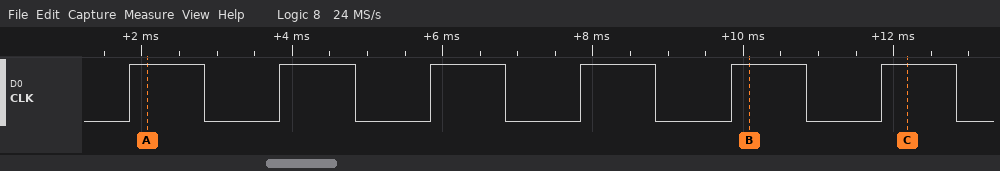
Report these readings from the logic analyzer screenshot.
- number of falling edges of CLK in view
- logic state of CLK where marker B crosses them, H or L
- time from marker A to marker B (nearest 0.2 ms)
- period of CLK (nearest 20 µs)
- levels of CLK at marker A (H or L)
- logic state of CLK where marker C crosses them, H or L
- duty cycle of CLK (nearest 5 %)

6
CLK=H
8 ms
2000 µs
CLK=H
CLK=H
50 %
